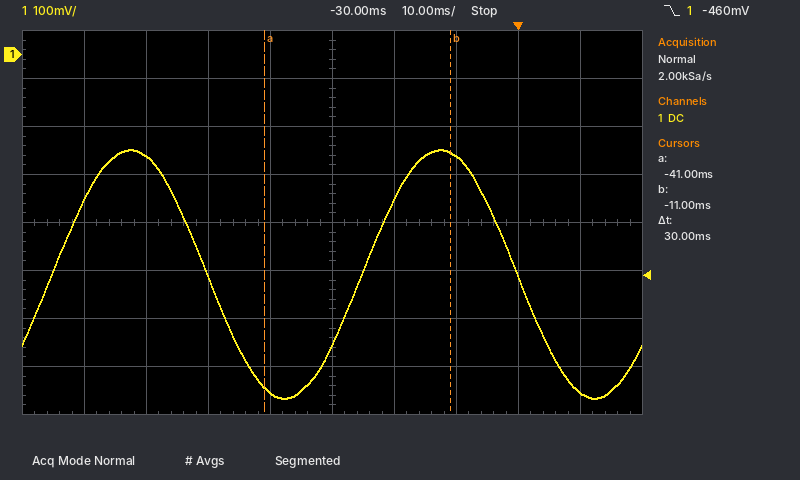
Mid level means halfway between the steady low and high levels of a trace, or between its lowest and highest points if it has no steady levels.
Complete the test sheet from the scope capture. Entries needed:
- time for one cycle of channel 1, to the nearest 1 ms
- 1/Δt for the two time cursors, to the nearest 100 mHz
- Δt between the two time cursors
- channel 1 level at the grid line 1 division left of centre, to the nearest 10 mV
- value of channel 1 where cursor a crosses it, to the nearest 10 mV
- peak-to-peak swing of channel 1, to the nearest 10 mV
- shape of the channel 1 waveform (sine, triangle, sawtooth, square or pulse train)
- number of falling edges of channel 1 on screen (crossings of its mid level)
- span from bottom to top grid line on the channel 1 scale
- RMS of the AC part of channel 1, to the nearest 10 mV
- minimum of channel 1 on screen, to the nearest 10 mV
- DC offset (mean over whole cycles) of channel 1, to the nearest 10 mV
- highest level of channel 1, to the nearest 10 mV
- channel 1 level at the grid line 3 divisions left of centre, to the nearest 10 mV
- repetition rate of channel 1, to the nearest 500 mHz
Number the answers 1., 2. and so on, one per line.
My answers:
1. 50 ms
2. 33.3 Hz
3. 30 ms
4. -700 mV
5. -690 mV
6. 520 mV
7. sine
8. 2
9. 800 mV
10. 180 mV
11. -720 mV
12. -460 mV
13. -200 mV
14. -210 mV
15. 20.0 Hz
